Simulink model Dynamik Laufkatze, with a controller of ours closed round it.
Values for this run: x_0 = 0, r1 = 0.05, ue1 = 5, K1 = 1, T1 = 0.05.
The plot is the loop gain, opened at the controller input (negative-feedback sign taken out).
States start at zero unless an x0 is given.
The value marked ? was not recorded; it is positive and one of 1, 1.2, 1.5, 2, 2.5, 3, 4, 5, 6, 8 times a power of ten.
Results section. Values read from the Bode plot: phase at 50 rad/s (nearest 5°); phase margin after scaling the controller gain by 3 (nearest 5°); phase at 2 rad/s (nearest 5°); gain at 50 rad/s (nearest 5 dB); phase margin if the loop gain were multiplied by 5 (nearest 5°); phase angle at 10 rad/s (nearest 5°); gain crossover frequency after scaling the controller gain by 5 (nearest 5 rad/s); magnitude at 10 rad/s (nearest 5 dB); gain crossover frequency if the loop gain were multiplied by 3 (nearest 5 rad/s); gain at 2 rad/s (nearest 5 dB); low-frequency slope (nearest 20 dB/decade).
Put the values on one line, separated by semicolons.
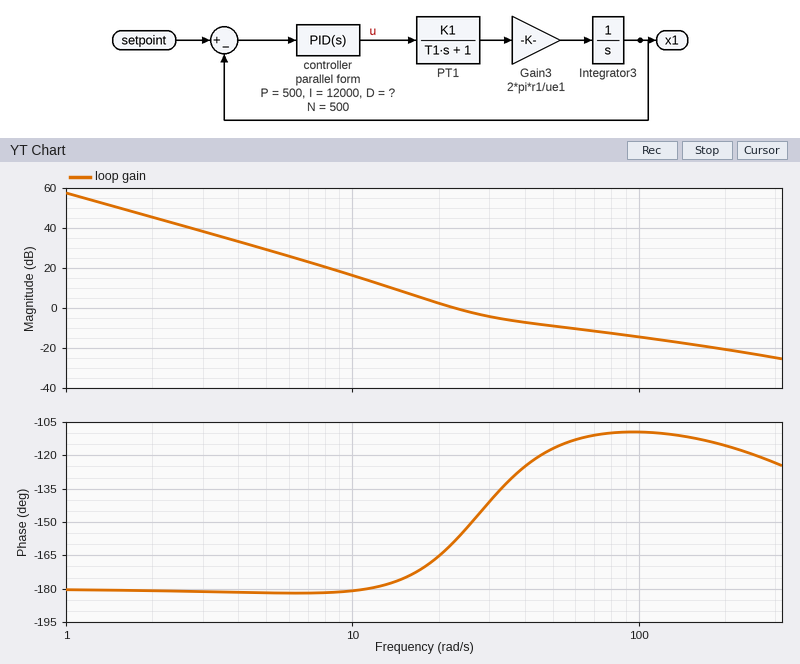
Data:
-115°; 65°; -180°; -10 dB; 70°; -180°; 95 rad/s; 15 dB; 55 rad/s; 45 dB; -40 dB/decade
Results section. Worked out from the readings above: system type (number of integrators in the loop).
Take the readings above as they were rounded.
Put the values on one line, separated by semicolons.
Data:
2
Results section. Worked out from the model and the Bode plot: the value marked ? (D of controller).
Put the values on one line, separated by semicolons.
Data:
15
